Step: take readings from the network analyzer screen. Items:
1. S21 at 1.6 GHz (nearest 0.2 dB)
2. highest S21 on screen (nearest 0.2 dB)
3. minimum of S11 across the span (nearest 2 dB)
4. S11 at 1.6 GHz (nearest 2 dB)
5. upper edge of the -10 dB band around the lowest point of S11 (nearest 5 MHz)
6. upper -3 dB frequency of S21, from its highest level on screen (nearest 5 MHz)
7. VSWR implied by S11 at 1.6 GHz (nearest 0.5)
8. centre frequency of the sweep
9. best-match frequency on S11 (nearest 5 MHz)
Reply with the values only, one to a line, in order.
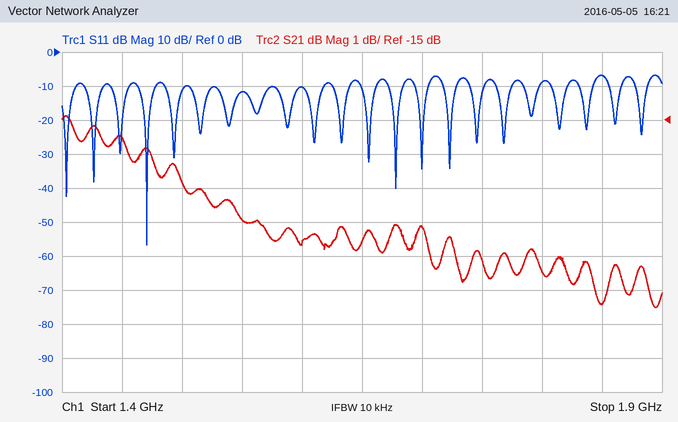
-18.6 dB
-14.8 dB
-56 dB
-10 dB
1.480 GHz
1.550 GHz
2.0
1.65 GHz
1.470 GHz
